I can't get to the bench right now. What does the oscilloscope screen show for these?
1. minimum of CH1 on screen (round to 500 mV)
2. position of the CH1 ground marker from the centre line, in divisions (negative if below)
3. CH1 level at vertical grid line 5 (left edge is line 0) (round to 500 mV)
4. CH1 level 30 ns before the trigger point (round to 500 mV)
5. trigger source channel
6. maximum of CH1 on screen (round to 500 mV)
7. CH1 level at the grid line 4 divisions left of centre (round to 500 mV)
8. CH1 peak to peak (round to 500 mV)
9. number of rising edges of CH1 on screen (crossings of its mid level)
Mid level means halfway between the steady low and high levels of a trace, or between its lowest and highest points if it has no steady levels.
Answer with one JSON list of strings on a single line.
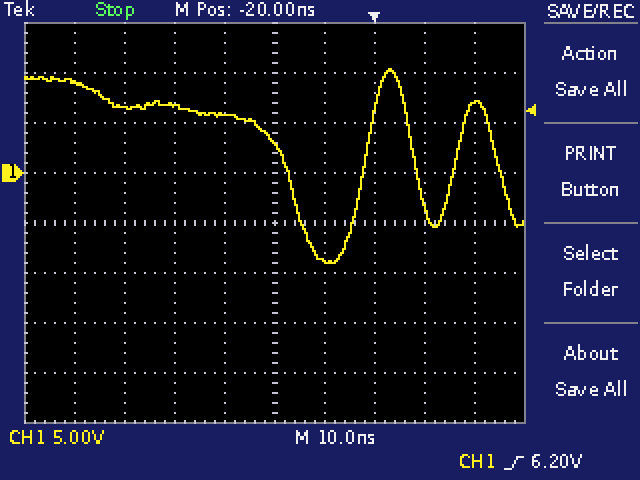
["-9.0 V", "+1.0 div", "3.0 V", "6.0 V", "CH1", "10.5 V", "9.0 V", "19.5 V", "2"]
